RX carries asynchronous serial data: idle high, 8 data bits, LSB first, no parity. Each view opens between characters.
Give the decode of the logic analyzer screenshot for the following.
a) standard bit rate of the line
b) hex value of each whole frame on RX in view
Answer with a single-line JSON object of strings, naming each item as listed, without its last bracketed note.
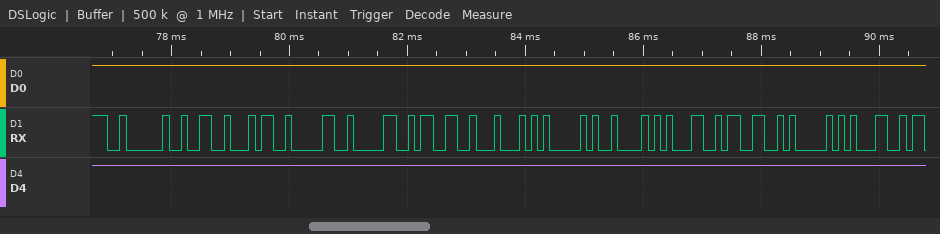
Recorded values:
{"standard bit rate of the line": "9600 baud", "hex value of each whole frame on RX in view": "02, 32, 34, 30, 30, 33, 44, 41, 42, 31, 33, 41, 31"}
